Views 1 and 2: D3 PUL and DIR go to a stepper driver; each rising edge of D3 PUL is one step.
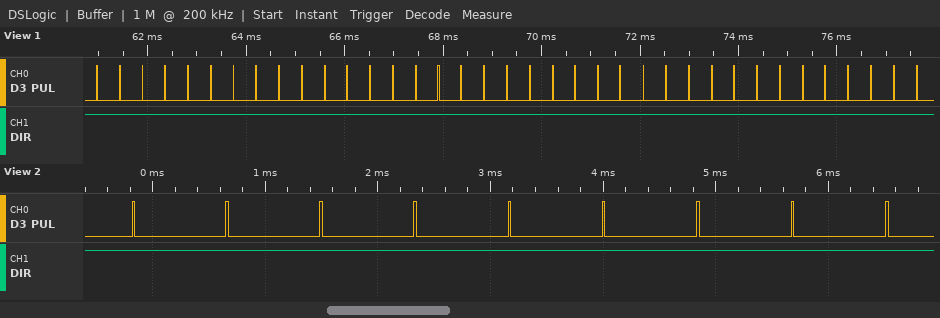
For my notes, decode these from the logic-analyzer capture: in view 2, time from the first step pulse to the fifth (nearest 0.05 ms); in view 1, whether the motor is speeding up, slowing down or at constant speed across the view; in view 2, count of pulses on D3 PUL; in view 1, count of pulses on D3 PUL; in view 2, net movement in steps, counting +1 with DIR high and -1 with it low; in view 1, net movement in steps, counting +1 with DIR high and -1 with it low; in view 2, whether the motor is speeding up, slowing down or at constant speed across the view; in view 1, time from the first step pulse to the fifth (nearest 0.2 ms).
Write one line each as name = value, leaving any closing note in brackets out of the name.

in view 2, time from the first step pulse to the fifth = 3.35 ms
in view 1, whether the motor is speeding up, slowing down or at constant speed across the view = constant speed
in view 2, count of pulses on D3 PUL = 9
in view 1, count of pulses on D3 PUL = 37
in view 2, net movement in steps, counting +1 with DIR high and -1 with it low = +9
in view 1, net movement in steps, counting +1 with DIR high and -1 with it low = +37
in view 2, whether the motor is speeding up, slowing down or at constant speed across the view = constant speed
in view 1, time from the first step pulse to the fifth = 1.8 ms
